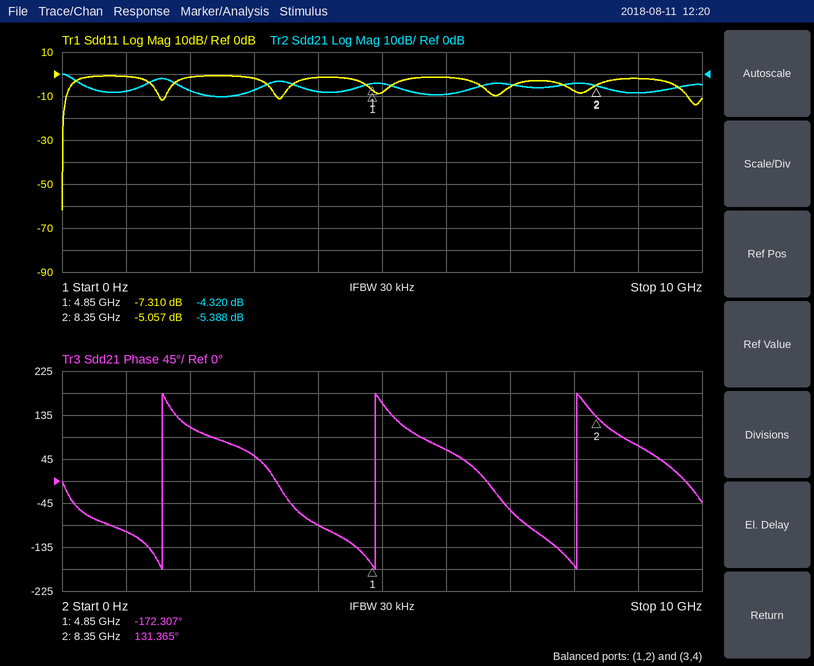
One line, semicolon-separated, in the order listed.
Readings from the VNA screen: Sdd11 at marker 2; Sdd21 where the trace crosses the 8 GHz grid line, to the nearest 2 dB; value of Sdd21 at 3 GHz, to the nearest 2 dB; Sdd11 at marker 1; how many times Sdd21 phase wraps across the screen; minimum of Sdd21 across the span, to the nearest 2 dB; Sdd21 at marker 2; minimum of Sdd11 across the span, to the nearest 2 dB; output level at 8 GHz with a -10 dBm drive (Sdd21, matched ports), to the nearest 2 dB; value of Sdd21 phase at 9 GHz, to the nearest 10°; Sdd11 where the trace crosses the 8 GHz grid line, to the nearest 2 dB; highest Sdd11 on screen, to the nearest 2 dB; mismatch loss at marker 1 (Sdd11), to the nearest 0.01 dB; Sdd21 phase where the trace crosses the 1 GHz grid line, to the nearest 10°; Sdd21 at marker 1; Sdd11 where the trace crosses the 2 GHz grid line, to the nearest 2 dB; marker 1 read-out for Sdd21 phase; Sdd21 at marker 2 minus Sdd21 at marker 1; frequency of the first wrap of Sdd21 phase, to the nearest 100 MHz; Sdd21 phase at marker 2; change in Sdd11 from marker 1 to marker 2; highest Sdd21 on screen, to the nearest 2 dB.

-5.057 dB; -4 dB; -8 dB; -7.310 dB; 3; -10 dB; -5.388 dB; -62 dB; -14 dBm; 70°; -8 dB; 0 dB; 0.89 dB; -100°; -4.320 dB; -2 dB; -172.307°; -1.068 dB; 1.6 GHz; 131.365°; 2.253 dB; 0 dB
